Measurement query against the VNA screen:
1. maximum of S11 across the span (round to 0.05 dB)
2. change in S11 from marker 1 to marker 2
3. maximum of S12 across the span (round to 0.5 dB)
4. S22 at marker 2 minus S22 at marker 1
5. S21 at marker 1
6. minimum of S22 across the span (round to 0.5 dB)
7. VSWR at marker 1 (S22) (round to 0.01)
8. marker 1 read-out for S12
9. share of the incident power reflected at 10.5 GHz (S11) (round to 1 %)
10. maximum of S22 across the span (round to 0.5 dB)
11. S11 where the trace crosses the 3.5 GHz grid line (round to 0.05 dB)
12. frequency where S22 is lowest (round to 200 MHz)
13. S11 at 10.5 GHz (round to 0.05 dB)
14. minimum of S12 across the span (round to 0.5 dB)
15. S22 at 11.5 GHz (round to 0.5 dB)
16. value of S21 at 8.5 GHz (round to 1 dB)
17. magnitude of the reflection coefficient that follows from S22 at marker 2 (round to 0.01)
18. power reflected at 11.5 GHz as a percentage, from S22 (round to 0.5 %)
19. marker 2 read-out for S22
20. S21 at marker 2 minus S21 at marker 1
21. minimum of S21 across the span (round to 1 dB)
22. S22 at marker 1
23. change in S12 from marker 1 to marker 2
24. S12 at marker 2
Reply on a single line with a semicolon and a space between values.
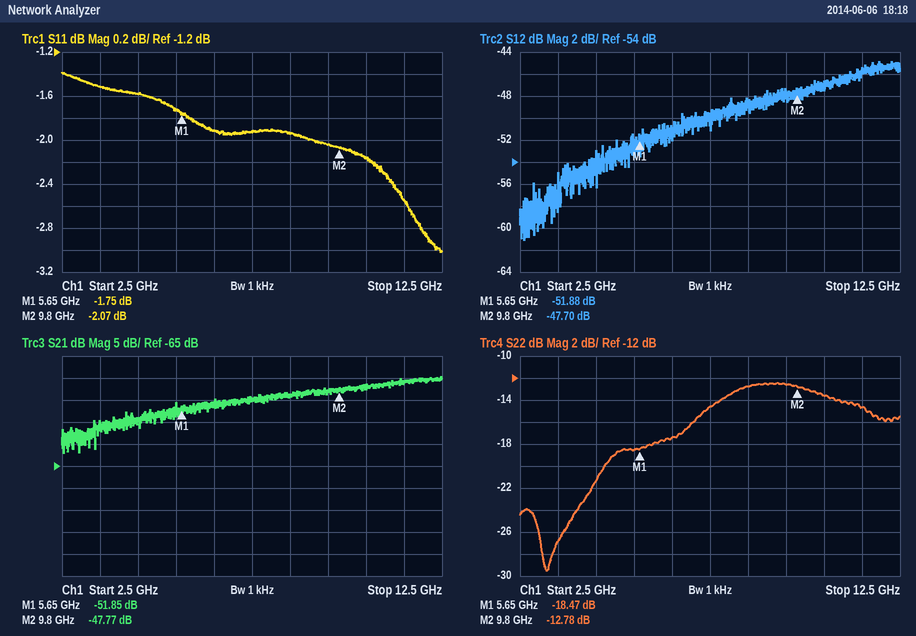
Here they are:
-1.40 dB; -0.32 dB; -45.0 dB; 5.69 dB; -51.85 dB; -29.5 dB; 1.27; -51.88 dB; 61 %; -12.5 dB; -1.50 dB; 3.2 GHz; -2.15 dB; -61.0 dB; -14.5 dB; -49 dB; 0.23; 3.5 %; -12.78 dB; 4.08 dB; -62 dB; -18.47 dB; 4.18 dB; -47.70 dB
